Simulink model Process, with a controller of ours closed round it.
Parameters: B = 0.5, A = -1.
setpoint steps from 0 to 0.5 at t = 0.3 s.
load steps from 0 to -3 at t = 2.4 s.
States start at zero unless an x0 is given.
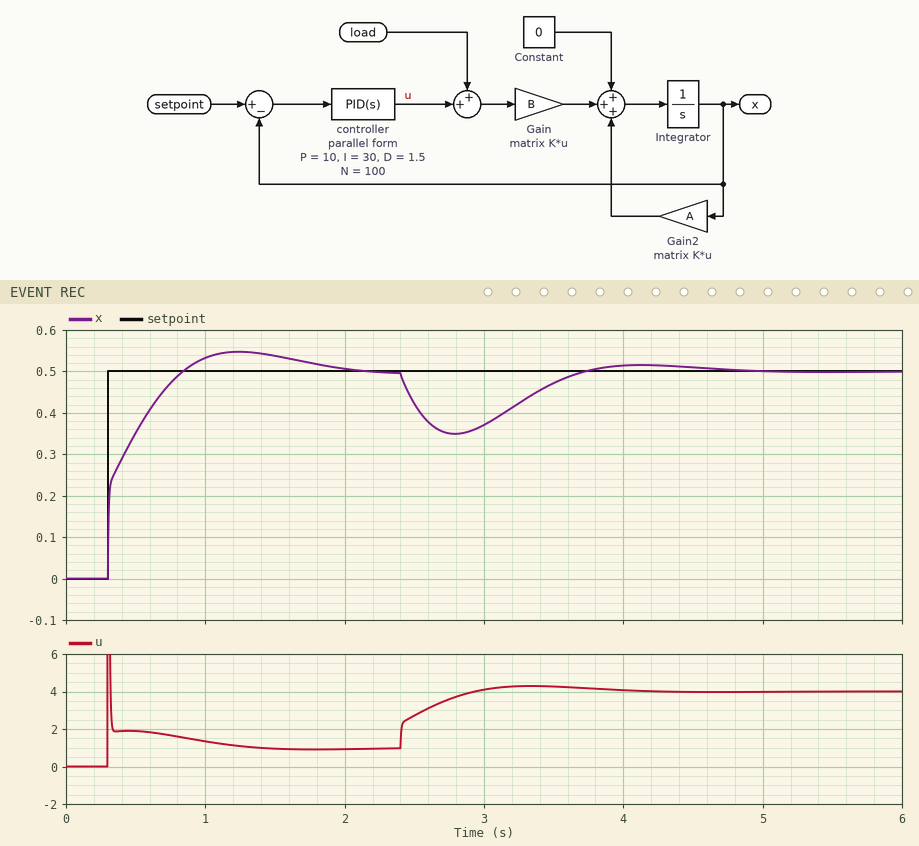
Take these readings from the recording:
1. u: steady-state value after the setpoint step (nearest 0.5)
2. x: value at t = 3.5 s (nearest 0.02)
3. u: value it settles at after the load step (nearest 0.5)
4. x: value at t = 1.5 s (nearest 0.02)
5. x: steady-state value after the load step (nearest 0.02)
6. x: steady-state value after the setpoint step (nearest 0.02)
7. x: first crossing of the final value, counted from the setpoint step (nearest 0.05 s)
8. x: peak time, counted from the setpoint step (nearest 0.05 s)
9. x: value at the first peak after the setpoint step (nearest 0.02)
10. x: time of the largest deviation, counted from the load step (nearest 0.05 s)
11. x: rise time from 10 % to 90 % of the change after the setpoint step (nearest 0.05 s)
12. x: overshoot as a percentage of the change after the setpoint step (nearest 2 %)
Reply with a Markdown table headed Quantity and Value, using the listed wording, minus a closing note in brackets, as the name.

| Quantity | Value |
|---|---|
| u: steady-state value after the setpoint step | 1.0 |
| x: value at t = 3.5 s | 0.48 |
| u: value it settles at after the load step | 4.0 |
| x: value at t = 1.5 s | 0.54 |
| x: steady-state value after the load step | 0.50 |
| x: steady-state value after the setpoint step | 0.50 |
| x: first crossing of the final value, counted from the setpoint step | 0.55 s |
| x: peak time, counted from the setpoint step | 0.95 s |
| x: value at the first peak after the setpoint step | 0.54 |
| x: time of the largest deviation, counted from the load step | 0.40 s |
| x: rise time from 10 % to 90 % of the change after the setpoint step | 0.40 s |
| x: overshoot as a percentage of the change after the setpoint step | 10 % |
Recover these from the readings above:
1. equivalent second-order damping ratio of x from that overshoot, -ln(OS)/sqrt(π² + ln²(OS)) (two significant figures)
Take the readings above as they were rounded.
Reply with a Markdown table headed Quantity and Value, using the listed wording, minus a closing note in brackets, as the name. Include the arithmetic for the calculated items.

| Quantity | Value |
|---|---|
| equivalent second-order damping ratio of x from that overshoot, -ln(OS)/sqrt(π² + ln²(OS)) | ln(0.1) = -2.303; 2.303 / sqrt(9.870 + 5.302) = 0.59 |
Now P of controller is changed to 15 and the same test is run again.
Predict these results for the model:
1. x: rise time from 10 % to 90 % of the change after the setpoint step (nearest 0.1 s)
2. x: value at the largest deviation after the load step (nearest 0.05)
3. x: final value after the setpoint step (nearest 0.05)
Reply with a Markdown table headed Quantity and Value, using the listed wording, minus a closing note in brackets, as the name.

| Quantity | Value |
|---|---|
| x: rise time from 10 % to 90 % of the change after the setpoint step | 0.3 s |
| x: value at the largest deviation after the load step | 0.40 |
| x: final value after the setpoint step | 0.50 |
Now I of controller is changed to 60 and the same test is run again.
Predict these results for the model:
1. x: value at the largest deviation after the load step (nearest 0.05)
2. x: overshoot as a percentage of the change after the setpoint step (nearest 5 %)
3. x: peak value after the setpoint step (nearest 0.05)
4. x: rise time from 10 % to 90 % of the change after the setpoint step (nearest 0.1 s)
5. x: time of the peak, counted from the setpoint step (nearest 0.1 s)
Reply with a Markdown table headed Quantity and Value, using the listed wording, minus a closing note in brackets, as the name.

| Quantity | Value |
|---|---|
| x: value at the largest deviation after the load step | 0.40 |
| x: overshoot as a percentage of the change after the setpoint step | 15 % |
| x: peak value after the setpoint step | 0.60 |
| x: rise time from 10 % to 90 % of the change after the setpoint step | 0.3 s |
| x: time of the peak, counted from the setpoint step | 0.7 s |
